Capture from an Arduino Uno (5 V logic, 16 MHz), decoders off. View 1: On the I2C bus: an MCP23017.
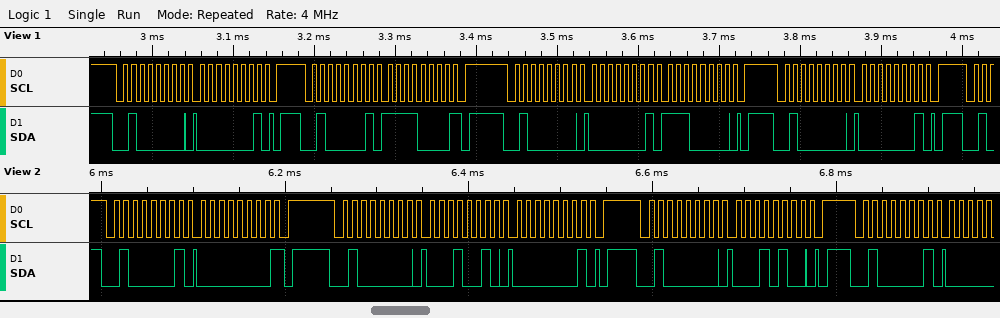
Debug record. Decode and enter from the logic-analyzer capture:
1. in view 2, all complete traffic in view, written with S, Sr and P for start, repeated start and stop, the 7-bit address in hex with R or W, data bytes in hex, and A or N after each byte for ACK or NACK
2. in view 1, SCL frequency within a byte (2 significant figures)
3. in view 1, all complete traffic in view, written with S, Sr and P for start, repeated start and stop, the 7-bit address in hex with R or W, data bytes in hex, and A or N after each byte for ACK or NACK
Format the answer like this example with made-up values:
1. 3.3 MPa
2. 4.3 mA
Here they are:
1. S 20R A 00 N P S 20W A 12 A 01 A P S 20W A 14 A P S 20R A
2. 100 kHz
3. S 20W A 01 A P S 20R A F0 N P S 20W A 01 A E0 A P S 20W A 01 A P
